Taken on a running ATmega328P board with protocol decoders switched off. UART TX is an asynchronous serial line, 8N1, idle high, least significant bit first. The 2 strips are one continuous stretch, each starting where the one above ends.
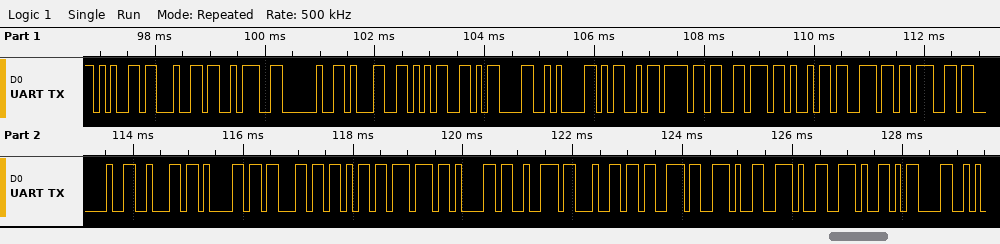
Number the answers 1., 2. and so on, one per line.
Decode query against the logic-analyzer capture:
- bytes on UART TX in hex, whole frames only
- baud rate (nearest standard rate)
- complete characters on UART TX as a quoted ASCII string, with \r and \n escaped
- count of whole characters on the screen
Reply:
1. 65 64 3A 20 31 35 0D 0A 4D 6F 76 69 6E 67 20 62 61 63 6B 77 61 72 64 73 2E 2E 2E 0D
2. 9600 baud
3. "ed: 15\r\nMoving backwards...\r"
4. 28
